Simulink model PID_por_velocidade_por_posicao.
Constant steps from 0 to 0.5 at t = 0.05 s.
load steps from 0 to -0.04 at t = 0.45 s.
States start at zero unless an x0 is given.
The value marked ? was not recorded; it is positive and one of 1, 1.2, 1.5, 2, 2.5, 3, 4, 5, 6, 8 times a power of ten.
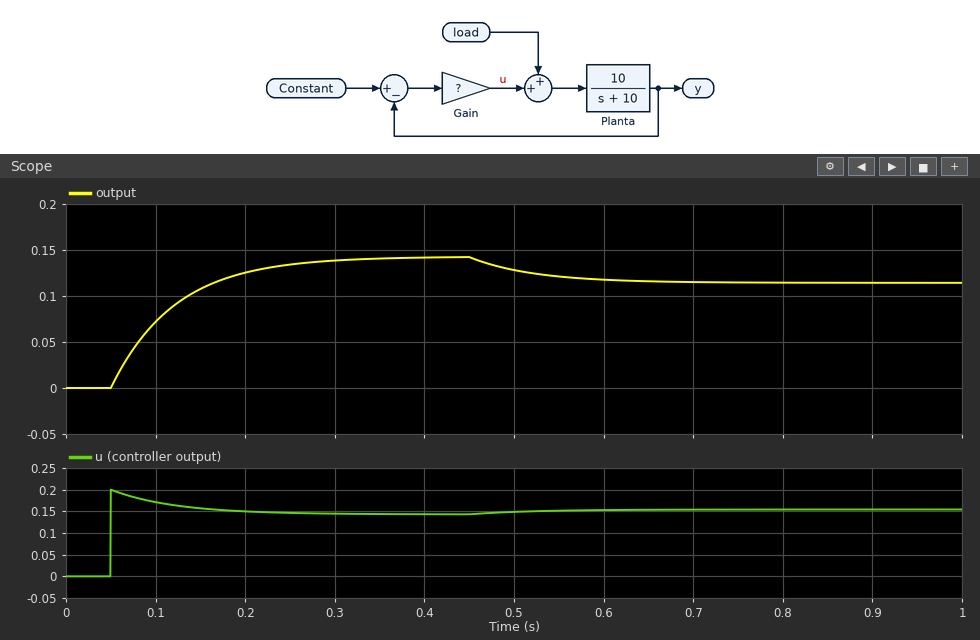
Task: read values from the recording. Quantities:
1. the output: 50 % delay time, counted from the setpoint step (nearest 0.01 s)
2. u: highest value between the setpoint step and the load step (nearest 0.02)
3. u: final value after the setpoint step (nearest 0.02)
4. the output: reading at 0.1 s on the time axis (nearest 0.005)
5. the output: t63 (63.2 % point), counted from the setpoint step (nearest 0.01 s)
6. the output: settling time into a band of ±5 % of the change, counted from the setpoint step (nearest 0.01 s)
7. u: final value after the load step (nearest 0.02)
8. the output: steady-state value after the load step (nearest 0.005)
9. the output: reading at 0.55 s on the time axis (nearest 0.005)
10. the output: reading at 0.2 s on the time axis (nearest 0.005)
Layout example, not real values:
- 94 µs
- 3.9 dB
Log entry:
- 0.05 s
- 0.20
- 0.14
- 0.070
- 0.07 s
- 0.21 s
- 0.16
- 0.115
- 0.120
- 0.125
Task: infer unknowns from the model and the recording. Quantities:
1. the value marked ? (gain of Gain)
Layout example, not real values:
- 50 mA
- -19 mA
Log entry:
- 0.4
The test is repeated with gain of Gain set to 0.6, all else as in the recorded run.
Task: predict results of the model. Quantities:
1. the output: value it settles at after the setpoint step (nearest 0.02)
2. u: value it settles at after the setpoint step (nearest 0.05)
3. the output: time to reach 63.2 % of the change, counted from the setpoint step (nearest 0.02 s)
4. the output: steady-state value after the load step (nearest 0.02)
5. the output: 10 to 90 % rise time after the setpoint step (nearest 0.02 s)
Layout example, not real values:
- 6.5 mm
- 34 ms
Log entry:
- 0.18
- 0.20
- 0.06 s
- 0.16
- 0.14 s
